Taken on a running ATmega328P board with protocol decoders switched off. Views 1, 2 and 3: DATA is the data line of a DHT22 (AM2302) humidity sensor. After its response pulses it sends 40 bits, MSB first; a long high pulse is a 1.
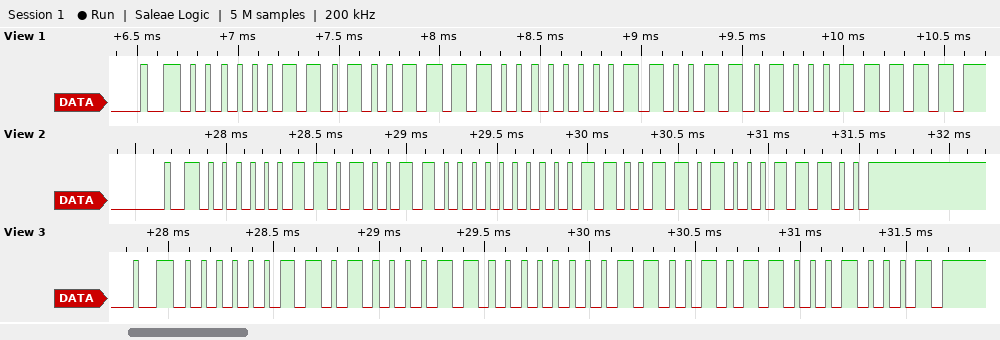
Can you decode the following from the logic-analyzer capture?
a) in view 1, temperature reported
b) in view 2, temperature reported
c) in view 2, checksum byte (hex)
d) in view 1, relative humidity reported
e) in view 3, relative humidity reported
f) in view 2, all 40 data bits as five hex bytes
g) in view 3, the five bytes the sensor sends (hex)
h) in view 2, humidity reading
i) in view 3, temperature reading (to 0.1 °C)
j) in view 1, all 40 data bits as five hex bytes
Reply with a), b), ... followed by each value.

a) 20.5 °C
b) 20.5 °C
c) 0x1C
d) 84.7 %
e) 83.5 %
f) 03 4C 00 CD 1C
g) 03 43 00 CB 11
h) 84.4 %
i) 20.3 °C
j) 03 4F 00 CD 1F
